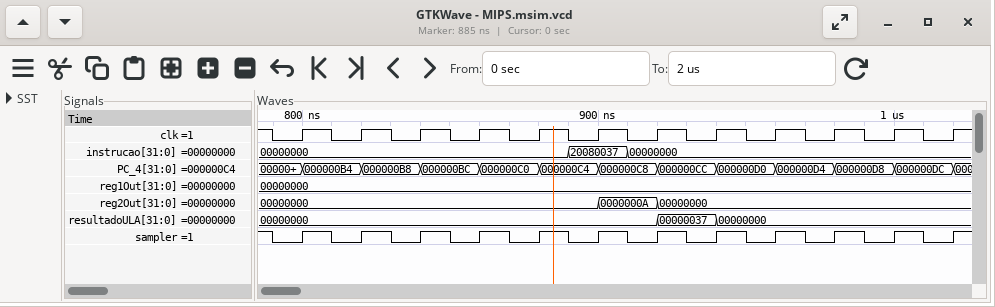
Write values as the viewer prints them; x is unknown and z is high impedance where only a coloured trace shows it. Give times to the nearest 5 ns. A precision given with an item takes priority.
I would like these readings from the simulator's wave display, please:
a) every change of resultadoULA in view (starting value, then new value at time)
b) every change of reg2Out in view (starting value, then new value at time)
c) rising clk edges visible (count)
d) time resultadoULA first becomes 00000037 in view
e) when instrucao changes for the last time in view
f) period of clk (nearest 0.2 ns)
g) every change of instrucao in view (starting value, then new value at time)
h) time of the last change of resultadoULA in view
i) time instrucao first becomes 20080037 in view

00000000, 00000037 at 920 ns, 00000000 at 940 ns
00000000, 0000000A at 900 ns, 00000000 at 920 ns
12
920 ns
910 ns
20 ns
00000000, 20080037 at 890 ns, 00000000 at 910 ns
940 ns
890 ns
